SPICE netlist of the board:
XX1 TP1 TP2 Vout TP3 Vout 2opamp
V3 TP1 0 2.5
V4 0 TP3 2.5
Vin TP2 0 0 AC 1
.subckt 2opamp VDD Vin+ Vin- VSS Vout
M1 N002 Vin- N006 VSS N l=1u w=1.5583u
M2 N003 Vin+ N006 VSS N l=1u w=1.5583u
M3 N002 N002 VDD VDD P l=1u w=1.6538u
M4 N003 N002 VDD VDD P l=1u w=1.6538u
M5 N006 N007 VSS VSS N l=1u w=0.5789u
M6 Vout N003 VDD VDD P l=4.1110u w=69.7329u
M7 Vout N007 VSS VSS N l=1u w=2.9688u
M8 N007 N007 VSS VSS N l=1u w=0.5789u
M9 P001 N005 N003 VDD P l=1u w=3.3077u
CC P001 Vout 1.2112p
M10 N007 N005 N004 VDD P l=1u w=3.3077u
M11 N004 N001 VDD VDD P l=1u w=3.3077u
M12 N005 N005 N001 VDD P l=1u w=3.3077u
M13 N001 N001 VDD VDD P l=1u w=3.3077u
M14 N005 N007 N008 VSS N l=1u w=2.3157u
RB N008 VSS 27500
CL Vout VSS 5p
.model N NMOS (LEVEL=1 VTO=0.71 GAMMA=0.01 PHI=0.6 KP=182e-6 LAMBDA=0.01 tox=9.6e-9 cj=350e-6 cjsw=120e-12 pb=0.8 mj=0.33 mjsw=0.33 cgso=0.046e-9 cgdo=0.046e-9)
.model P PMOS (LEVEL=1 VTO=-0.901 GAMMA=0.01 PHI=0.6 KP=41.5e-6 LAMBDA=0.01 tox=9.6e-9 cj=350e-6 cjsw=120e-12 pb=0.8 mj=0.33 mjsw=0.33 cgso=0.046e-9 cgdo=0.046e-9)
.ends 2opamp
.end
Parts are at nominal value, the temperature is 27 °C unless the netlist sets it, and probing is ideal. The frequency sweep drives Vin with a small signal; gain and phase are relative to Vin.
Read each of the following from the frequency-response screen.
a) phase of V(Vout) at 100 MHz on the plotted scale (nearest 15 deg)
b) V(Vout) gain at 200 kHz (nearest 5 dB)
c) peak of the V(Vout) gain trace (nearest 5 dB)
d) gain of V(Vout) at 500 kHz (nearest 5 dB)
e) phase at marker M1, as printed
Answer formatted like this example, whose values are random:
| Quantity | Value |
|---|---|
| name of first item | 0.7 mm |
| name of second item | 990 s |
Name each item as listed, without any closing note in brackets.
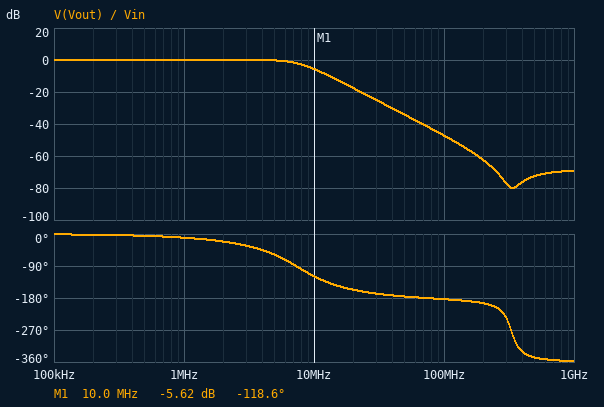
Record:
| Quantity | Value |
|---|---|
| phase of V(Vout) at 100 MHz on the plotted scale | -180 deg |
| V(Vout) gain at 200 kHz | 0 dB |
| peak of the V(Vout) gain trace | 0 dB |
| gain of V(Vout) at 500 kHz | 0 dB |
| phase at marker M1, as printed | -118.6 deg |
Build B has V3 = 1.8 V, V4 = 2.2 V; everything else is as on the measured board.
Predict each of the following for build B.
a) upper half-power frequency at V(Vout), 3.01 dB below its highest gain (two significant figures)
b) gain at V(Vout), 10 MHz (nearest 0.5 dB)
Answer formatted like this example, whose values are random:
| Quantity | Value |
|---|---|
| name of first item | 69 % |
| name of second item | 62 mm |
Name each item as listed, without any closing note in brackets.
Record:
| Quantity | Value |
|---|---|
| upper half-power frequency at V(Vout), 3.01 dB below its highest gain | 8.0 MHz |
| gain at V(Vout), 10 MHz | -6.0 dB |
